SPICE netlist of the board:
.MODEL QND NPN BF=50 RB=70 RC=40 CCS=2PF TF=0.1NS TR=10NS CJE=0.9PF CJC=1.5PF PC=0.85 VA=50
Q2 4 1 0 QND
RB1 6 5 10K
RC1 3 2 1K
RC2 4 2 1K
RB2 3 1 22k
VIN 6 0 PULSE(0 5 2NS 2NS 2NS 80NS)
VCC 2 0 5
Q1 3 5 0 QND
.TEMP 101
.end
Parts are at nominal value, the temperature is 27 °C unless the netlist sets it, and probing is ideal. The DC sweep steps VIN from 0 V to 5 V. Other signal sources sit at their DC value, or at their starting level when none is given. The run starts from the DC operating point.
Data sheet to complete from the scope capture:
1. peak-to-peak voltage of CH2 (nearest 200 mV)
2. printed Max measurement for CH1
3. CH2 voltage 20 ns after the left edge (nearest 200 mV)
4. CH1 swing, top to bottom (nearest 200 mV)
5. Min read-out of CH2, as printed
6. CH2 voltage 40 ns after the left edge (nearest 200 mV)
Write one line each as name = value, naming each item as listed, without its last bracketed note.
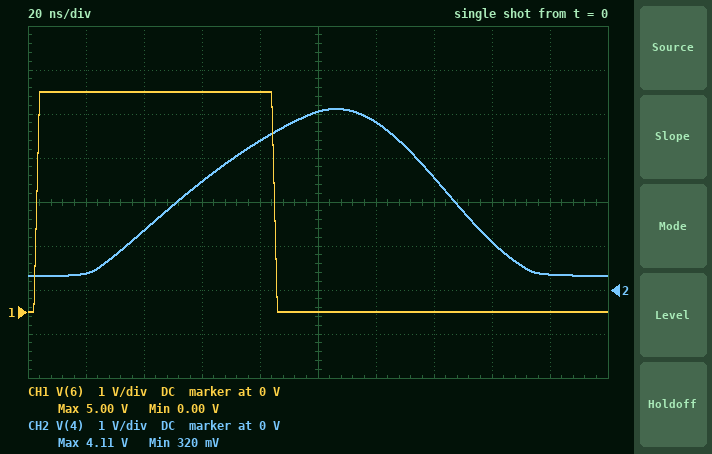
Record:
peak-to-peak voltage of CH2 = 3.8 V
printed Max measurement for CH1 = 5.00 V
CH2 voltage 20 ns after the left edge = 400 mV
CH1 swing, top to bottom = 5.0 V
Min read-out of CH2, as printed = 320 mV
CH2 voltage 40 ns after the left edge = 1.4 V
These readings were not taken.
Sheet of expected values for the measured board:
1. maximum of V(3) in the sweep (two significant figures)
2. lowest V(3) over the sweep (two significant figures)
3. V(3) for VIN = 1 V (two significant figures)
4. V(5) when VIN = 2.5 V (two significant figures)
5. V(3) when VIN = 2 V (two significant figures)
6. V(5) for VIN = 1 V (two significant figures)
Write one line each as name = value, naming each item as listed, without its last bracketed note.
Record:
maximum of V(3) in the sweep = 4.8 V
lowest V(3) over the sweep = 280 mV
V(3) for VIN = 1 V = 3.2 V
V(5) when VIN = 2.5 V = 730 mV
V(3) when VIN = 2 V = 350 mV
V(5) for VIN = 1 V = 690 mV
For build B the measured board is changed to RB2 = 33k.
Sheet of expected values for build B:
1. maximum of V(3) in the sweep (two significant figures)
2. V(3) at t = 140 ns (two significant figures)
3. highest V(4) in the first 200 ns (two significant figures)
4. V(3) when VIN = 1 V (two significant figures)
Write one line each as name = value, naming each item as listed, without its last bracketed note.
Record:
maximum of V(3) in the sweep = 4.9 V
V(3) at t = 140 ns = 3.9 V
highest V(4) in the first 200 ns = 4.0 V
V(3) when VIN = 1 V = 3.3 V
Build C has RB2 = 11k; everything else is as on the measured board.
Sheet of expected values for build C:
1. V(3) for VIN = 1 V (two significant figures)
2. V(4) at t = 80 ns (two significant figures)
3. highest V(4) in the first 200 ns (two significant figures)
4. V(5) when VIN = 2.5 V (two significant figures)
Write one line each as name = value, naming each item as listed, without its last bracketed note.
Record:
V(3) for VIN = 1 V = 3.1 V
V(4) at t = 80 ns = 3.7 V
highest V(4) in the first 200 ns = 4.5 V
V(5) when VIN = 2.5 V = 730 mV
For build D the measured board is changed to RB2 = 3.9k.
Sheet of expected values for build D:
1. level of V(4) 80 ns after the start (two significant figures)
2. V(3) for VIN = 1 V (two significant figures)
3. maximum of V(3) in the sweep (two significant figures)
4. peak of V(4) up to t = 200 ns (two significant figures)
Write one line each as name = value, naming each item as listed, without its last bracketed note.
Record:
level of V(4) 80 ns after the start = 4.9 V
V(3) for VIN = 1 V = 2.8 V
maximum of V(3) in the sweep = 4.1 V
peak of V(4) up to t = 200 ns = 5.0 V
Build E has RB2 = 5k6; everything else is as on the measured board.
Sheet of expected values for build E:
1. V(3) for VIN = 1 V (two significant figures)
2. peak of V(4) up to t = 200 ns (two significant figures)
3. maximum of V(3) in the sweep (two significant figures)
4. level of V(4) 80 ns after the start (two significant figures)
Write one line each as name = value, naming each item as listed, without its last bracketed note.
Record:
V(3) for VIN = 1 V = 3.0 V
peak of V(4) up to t = 200 ns = 5.0 V
maximum of V(3) in the sweep = 4.4 V
level of V(4) 80 ns after the start = 4.5 V
